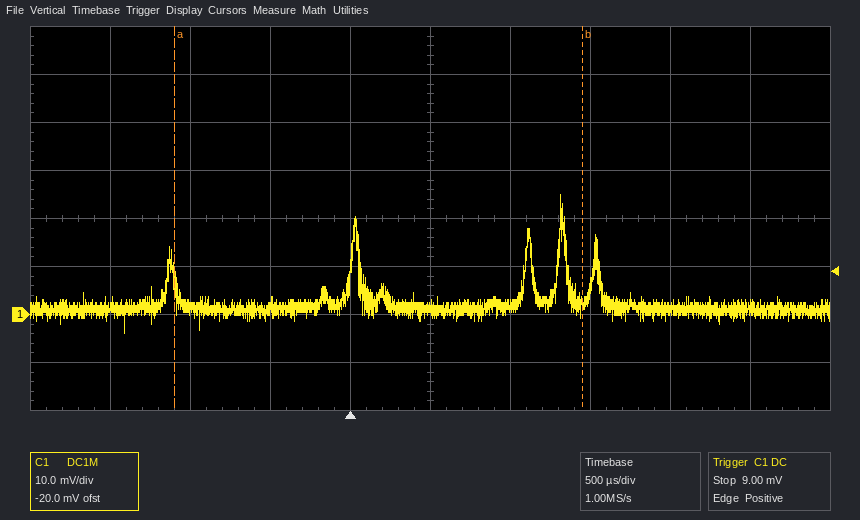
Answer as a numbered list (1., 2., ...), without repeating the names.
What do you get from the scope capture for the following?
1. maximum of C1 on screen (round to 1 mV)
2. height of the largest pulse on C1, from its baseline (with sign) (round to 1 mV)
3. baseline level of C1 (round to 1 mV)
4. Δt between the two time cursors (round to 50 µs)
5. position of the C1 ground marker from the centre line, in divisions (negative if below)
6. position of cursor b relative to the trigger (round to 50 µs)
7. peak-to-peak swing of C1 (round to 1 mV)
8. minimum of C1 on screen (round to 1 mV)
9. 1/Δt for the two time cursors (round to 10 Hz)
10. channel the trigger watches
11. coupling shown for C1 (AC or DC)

1. 25 mV
2. +24 mV
3. 1 mV
4. 2.55 ms
5. -2.0 div
6. +1.45 ms
7. 29 mV
8. -4 mV
9. 390 Hz
10. C1
11. DC
